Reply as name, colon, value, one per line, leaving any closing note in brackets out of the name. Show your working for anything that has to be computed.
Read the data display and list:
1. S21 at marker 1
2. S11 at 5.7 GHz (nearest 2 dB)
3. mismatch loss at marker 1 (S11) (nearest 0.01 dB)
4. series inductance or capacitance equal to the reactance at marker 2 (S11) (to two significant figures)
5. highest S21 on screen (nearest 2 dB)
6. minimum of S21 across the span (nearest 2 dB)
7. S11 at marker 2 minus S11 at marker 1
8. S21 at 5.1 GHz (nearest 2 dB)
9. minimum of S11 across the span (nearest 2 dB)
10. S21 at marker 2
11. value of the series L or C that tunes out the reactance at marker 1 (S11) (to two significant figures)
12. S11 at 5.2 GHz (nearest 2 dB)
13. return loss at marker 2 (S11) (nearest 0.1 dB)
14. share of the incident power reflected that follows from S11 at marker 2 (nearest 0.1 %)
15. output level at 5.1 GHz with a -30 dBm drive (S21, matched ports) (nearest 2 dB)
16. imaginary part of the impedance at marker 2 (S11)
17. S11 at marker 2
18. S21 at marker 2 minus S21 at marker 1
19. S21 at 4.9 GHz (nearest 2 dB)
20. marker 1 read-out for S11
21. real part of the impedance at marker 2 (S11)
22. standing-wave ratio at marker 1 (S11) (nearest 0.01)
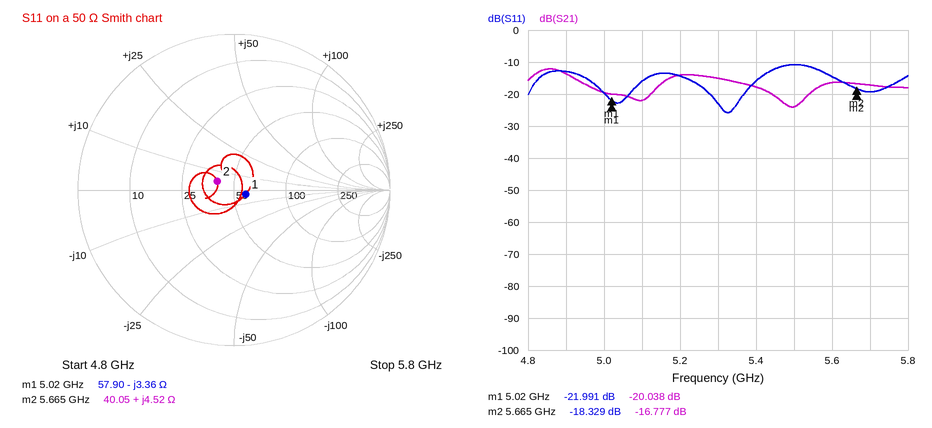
S21 at marker 1: -20.038 dB
S11 at 5.7 GHz: -20 dB
mismatch loss at marker 1 (S11): −10 log10(1 − 10^(-21.991/10)) ≈ 0.03 dB
series inductance or capacitance equal to the reactance at marker 2 (S11): L = 4.52 Ω/(2π × 5.665 GHz) ≈ 127 pH, so 130 pH to two significant figures
highest S21 on screen: -12 dB
minimum of S21 across the span: -24 dB
S11 at marker 2 minus S11 at marker 1: -18.329 − (-21.991) = 3.662 dB
S21 at 5.1 GHz: -22 dB
minimum of S11 across the span: -26 dB
S21 at marker 2: -16.777 dB
value of the series L or C that tunes out the reactance at marker 1 (S11): L = 3.36 Ω/(2π × 5.02 GHz) ≈ 107 pH, so 110 pH to two significant figures
S11 at 5.2 GHz: -14 dB
return loss at marker 2 (S11): 18.3 dB
share of the incident power reflected that follows from S11 at marker 2: 10^(-18.329/10) ≈ 1.5 %
output level at 5.1 GHz with a -30 dBm drive (S21, matched ports): -30 dBm + (-22 dB) = -52 dBm
imaginary part of the impedance at marker 2: +4.52 Ω
S11 at marker 2: -18.329 dB
S21 at marker 2 minus S21 at marker 1: -16.777 − (-20.038) = 3.261 dB
S21 at 4.9 GHz: -14 dB
marker 1 read-out for S11: -21.991 dB
real part of the impedance at marker 2: 40.05 Ω
standing-wave ratio at marker 1 (S11): 1.17
